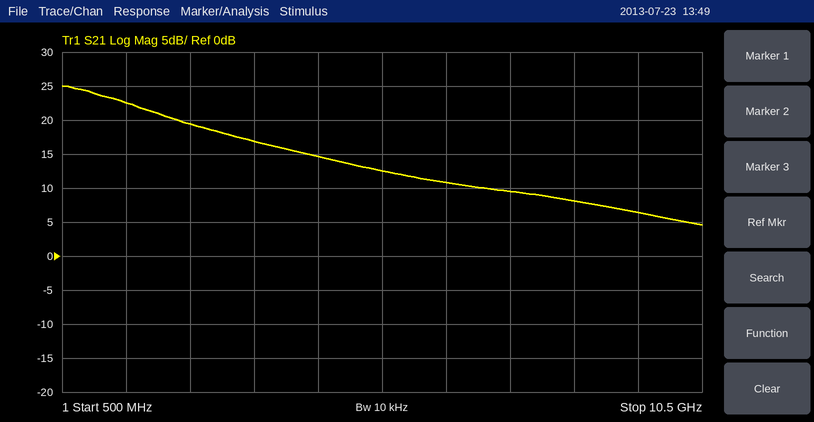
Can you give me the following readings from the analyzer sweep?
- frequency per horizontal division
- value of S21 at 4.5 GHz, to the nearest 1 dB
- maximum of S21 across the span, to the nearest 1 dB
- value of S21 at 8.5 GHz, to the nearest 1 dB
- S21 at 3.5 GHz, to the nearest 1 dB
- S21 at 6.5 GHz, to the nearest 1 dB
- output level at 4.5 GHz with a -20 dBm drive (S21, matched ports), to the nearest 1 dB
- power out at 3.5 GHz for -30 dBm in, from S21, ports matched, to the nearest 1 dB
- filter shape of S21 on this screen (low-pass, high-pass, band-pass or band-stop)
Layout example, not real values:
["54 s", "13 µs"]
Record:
["1 GHz", "15 dB", "25 dB", "8 dB", "17 dB", "11 dB", "-5 dBm", "-13 dBm", "low-pass"]
